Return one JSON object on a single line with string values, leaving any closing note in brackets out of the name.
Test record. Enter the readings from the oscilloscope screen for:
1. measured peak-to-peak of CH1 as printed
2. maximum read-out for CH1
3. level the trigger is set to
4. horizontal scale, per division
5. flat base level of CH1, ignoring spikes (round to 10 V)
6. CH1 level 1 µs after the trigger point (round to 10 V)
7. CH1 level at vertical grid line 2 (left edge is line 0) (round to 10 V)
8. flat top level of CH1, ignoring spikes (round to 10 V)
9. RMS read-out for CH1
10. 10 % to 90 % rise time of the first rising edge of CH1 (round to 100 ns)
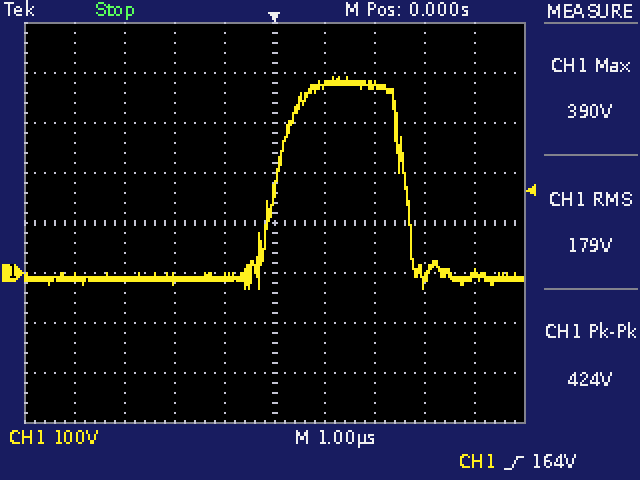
{"measured peak-to-peak of CH1 as printed": "424 V", "maximum read-out for CH1": "390 V", "level the trigger is set to": "164 V", "horizontal scale, per division": "1 µs", "flat base level of CH1, ignoring spikes": "-10 V", "CH1 level 1 µs after the trigger point": "380 V", "CH1 level at vertical grid line 2 (left edge is line 0)": "-10 V", "flat top level of CH1, ignoring spikes": "380 V", "RMS read-out for CH1": "179 V", "10 % to 90 % rise time of the first rising edge of CH1": "800 ns"}
